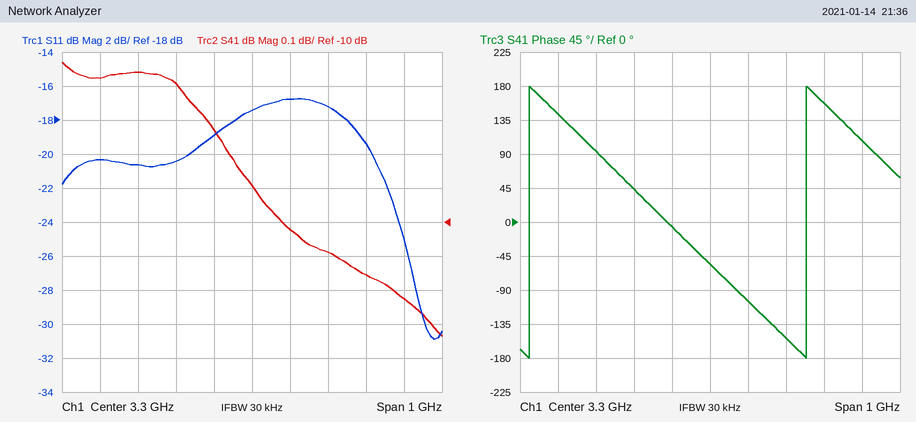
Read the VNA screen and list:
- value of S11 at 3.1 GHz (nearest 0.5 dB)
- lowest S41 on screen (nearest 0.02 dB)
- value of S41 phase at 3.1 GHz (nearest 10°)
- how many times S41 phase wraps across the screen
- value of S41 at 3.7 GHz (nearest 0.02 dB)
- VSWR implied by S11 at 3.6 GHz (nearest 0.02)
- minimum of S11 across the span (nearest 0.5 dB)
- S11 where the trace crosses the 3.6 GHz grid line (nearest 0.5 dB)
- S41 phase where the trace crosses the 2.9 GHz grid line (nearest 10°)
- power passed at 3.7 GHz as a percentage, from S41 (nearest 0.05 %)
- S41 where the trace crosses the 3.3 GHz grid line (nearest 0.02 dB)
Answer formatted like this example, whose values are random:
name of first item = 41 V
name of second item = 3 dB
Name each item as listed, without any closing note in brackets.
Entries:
value of S11 at 3.1 GHz = -20.5 dB
lowest S41 on screen = -10.34 dB
value of S41 phase at 3.1 GHz = 40°
how many times S41 phase wraps across the screen = 2
value of S41 at 3.7 GHz = -10.22 dB
VSWR implied by S11 at 3.6 GHz = 1.24
minimum of S11 across the span = -31.0 dB
S11 where the trace crosses the 3.6 GHz grid line = -19.5 dB
S41 phase where the trace crosses the 2.9 GHz grid line = 140°
power passed at 3.7 GHz as a percentage, from S41 = 9.50 %
S41 where the trace crosses the 3.3 GHz grid line = -9.90 dB
